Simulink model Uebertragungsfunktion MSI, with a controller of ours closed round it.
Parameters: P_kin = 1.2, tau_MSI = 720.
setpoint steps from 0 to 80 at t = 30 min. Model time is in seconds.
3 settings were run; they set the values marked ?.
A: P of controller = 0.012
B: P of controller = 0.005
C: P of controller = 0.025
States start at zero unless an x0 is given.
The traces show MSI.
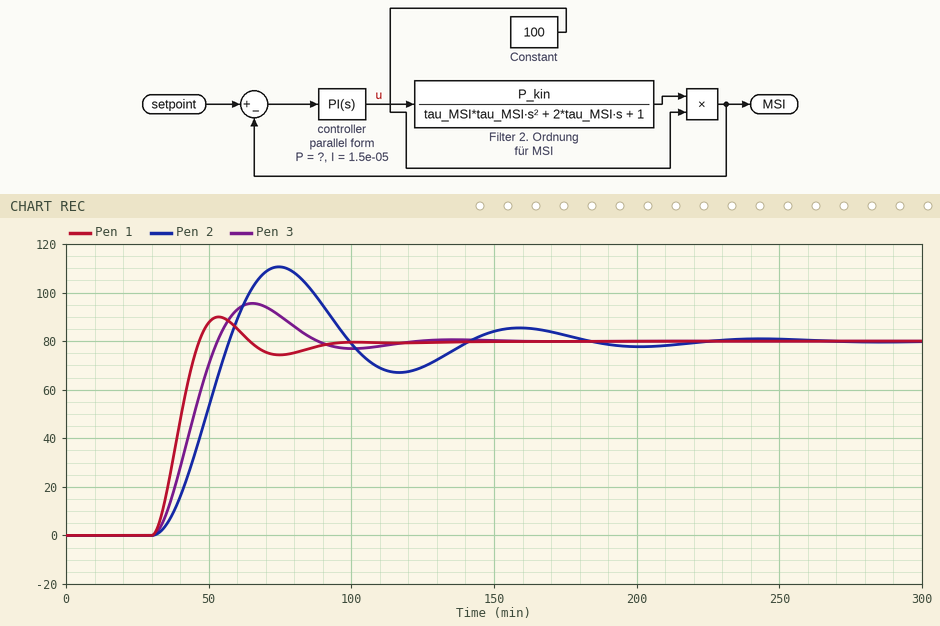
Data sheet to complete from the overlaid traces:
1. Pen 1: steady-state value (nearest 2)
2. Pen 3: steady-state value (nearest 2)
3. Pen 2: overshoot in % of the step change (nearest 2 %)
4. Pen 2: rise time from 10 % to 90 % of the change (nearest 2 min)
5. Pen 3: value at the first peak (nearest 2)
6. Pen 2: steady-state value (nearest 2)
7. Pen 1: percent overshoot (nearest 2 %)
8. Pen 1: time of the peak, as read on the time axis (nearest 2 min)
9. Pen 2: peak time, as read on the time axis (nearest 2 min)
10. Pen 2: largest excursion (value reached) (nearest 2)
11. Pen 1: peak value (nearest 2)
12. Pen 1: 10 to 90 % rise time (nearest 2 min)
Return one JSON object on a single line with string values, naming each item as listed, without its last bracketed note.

{"Pen 1: steady-state value": "80", "Pen 3: steady-state value": "80", "Pen 2: overshoot in % of the step change": "38 %", "Pen 2: rise time from 10 % to 90 % of the change": "18 min", "Pen 3: value at the first peak": "96", "Pen 2: steady-state value": "80", "Pen 1: percent overshoot": "12 %", "Pen 1: time of the peak, as read on the time axis": "54 min", "Pen 2: peak time, as read on the time axis": "74 min", "Pen 2: largest excursion (value reached)": "110", "Pen 1: peak value": "90", "Pen 1: 10 to 90 % rise time": "12 min"}
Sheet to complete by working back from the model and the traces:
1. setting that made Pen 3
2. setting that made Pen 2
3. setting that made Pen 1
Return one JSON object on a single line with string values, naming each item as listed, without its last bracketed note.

{"setting that made Pen 3": "A", "setting that made Pen 2": "B", "setting that made Pen 1": "C"}
